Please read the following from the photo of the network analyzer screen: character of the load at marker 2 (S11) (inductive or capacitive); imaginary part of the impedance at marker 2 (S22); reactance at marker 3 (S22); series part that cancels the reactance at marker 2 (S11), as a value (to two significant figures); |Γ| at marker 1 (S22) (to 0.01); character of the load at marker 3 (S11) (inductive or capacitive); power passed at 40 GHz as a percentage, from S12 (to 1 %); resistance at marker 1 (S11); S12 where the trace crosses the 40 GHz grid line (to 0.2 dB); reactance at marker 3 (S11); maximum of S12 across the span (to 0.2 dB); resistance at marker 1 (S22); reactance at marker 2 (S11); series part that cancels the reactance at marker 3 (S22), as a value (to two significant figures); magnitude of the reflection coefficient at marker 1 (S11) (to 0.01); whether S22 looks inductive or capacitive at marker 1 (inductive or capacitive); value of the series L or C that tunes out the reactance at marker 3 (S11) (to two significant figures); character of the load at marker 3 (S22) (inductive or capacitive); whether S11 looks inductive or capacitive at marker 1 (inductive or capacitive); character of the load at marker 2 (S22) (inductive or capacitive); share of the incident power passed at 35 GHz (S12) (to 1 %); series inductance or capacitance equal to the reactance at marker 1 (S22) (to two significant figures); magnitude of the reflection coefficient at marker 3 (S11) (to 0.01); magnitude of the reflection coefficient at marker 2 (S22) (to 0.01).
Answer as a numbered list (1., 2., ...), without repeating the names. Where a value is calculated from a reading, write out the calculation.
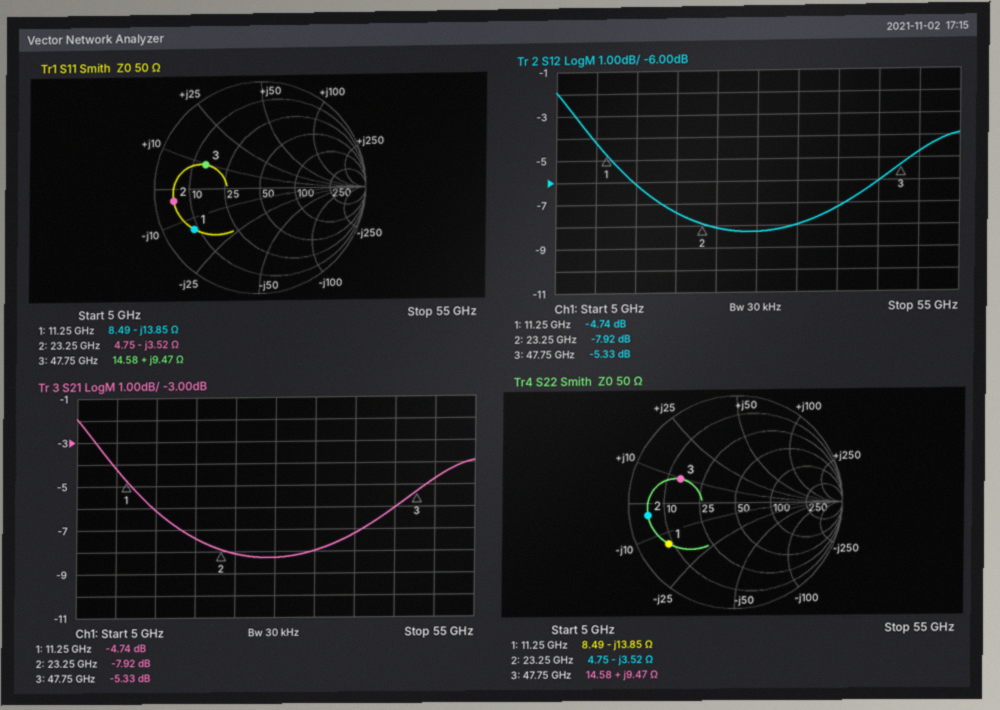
1. capacitive
2. -3.52 Ω
3. +9.47 Ω
4. L = 3.52 Ω/(2π × 23.25 GHz) ≈ 24 pH
5. 0.73
6. inductive
7. 10^(-7.2/10) ≈ 19 %
8. 8.49 Ω
9. -7.2 dB
10. +9.47 Ω
11. -2.0 dB
12. 8.49 Ω
13. -3.52 Ω
14. C = 1/(2π × 47.75 GHz × 9.47 Ω) ≈ 352 fF, so 350 fF to two significant figures
15. 0.73
16. capacitive
17. C = 1/(2π × 47.75 GHz × 9.47 Ω) ≈ 352 fF, so 350 fF to two significant figures
18. inductive
19. capacitive
20. capacitive
21. 10^(-8/10) ≈ 16 %
22. C = 1/(2π × 11.25 GHz × 13.85 Ω) ≈ 1.0 pF
23. 0.56
24. 0.83
